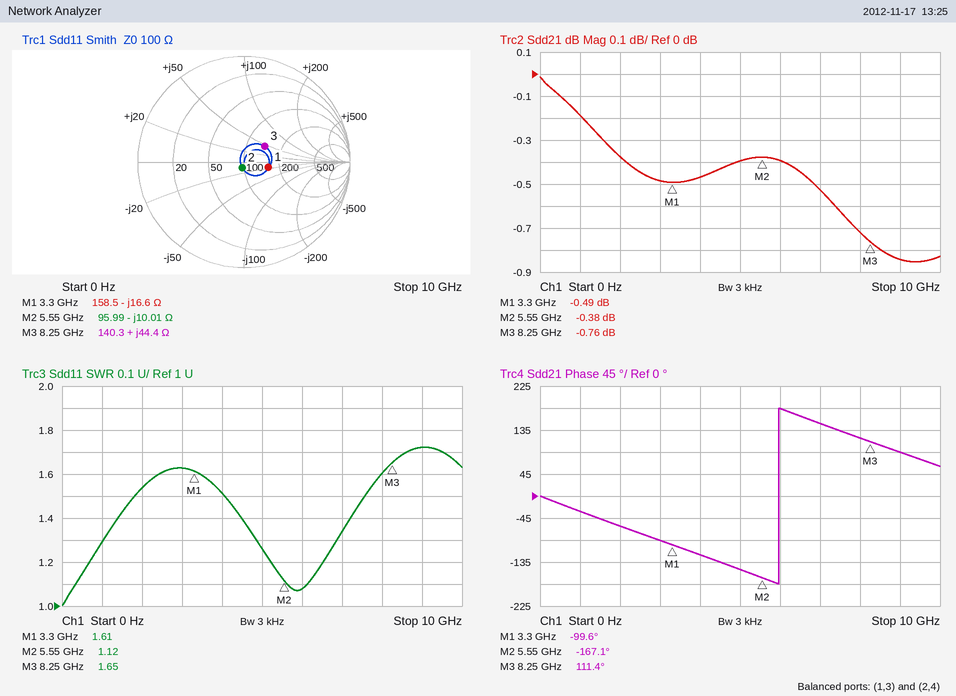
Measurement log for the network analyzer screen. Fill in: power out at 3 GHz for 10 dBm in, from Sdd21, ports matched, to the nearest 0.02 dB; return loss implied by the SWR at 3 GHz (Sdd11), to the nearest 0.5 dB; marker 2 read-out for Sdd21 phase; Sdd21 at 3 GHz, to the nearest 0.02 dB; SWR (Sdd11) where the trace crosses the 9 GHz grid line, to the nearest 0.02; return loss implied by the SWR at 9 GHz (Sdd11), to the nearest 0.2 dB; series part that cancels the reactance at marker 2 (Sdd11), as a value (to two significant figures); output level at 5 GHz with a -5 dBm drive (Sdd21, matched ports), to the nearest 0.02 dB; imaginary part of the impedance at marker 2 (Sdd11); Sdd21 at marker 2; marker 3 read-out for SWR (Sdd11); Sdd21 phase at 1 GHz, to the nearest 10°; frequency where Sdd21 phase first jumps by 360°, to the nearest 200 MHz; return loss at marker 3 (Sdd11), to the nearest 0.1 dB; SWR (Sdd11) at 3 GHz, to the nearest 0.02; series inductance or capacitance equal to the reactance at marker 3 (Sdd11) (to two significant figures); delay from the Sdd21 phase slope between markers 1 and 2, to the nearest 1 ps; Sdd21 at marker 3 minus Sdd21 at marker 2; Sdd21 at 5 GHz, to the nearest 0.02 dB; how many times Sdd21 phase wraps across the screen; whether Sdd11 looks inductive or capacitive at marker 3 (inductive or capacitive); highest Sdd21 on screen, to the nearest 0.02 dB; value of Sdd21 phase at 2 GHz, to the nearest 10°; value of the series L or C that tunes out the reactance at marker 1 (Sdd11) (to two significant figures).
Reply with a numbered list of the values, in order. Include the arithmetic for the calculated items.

1. 10 dBm + (-0.48 dB) = 9.52 dBm
2. −20 log10((1.62 − 1)/(1.62 + 1)) ≈ 12.5 dB
3. -167.1°
4. -0.48 dB
5. 1.72
6. −20 log10((1.72 − 1)/(1.72 + 1)) ≈ 11.5 dB, so 11.6 dB to the nearest 0.2 dB
7. L = 10.01 Ω/(2π × 5.55 GHz) ≈ 287 pH, so 290 pH to two significant figures
8. -5 dBm + (-0.40 dB) = -5.40 dBm
9. -10.01 Ω
10. -0.38 dB
11. 1.65
12. -30°
13. 6.0 GHz
14. 12.2 dB
15. 1.62
16. L = 44.4 Ω/(2π × 8.25 GHz) ≈ 857 pH, so 860 pH to two significant figures
17. −(-167.1° − (-99.6°))/(360° × 2.25 GHz) ≈ 83 ps
18. -0.76 − (-0.38) = -0.38 dB
19. -0.40 dB
20. 1
21. inductive
22. -0.02 dB
23. -60°
24. L = 16.6 Ω/(2π × 3.3 GHz) ≈ 801 pH, so 800 pH to two significant figures
